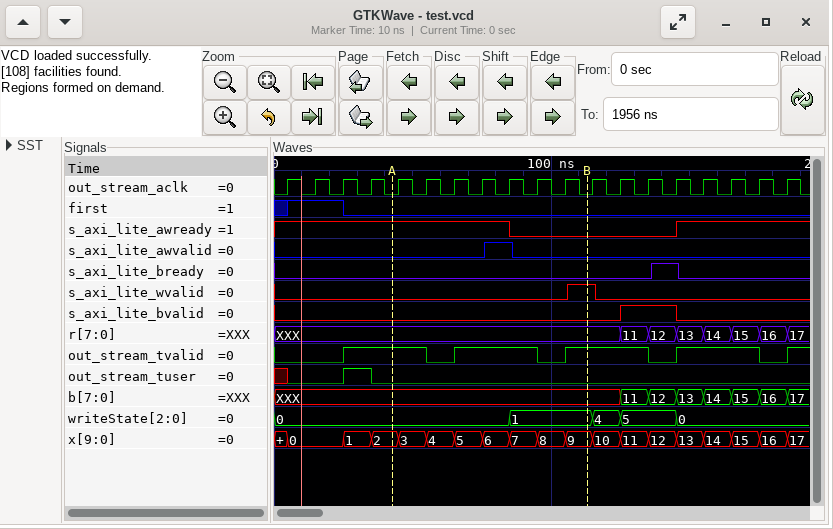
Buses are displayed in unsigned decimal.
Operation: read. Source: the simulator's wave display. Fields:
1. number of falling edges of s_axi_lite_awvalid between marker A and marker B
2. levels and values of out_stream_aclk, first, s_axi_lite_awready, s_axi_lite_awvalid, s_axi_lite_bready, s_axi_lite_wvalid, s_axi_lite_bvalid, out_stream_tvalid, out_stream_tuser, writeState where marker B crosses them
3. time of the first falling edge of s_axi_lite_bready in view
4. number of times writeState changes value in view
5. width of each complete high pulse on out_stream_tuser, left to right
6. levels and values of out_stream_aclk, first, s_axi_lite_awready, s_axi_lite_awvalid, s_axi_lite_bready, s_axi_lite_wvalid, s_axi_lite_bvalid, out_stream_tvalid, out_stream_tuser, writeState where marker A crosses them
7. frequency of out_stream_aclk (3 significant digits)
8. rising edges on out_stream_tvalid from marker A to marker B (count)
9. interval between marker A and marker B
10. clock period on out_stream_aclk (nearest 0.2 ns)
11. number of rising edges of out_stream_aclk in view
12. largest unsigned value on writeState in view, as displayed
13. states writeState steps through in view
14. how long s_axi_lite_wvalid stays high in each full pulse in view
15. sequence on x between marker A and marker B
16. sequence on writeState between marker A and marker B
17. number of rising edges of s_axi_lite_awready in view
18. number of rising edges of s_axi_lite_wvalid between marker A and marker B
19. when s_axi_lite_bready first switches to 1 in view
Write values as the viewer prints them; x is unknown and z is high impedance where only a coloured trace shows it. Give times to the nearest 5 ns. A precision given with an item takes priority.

1
out_stream_aclk=0, first=0, s_axi_lite_awready=0, s_axi_lite_awvalid=0, s_axi_lite_bready=0, s_axi_lite_wvalid=1, s_axi_lite_bvalid=0, out_stream_tvalid=1, out_stream_tuser=0, writeState=1
145 ns
4
10 ns
out_stream_aclk=0, first=0, s_axi_lite_awready=1, s_axi_lite_awvalid=0, s_axi_lite_bready=0, s_axi_lite_wvalid=0, s_axi_lite_bvalid=0, out_stream_tvalid=1, out_stream_tuser=0, writeState=0
100 MHz
2
70 ns
10 ns
19
5
0, 1, 4, 5, 0
10 ns
2, 3, 4, 5, 6, 7, 8, 9
0, 1
1
1
135 ns
